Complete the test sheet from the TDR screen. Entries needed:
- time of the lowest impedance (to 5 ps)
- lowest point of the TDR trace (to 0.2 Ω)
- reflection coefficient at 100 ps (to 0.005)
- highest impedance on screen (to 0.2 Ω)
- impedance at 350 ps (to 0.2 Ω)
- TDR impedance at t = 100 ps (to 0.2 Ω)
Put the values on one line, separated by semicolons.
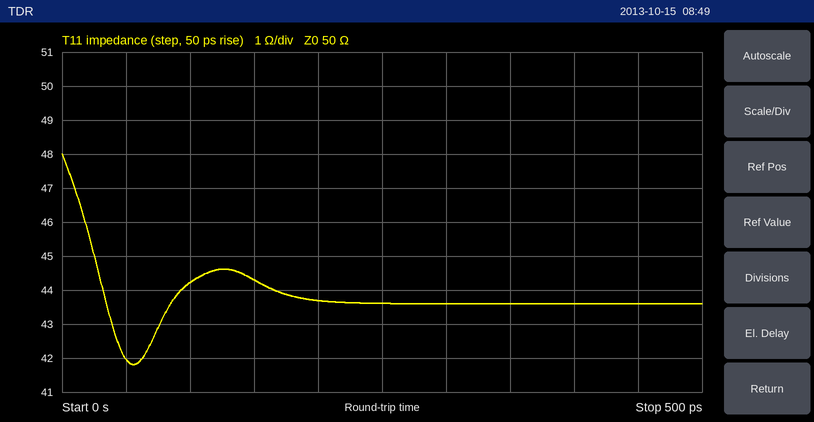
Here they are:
55 ps; 41.8 Ω; -0.060; 48.0 Ω; 43.6 Ω; 44.2 Ω
